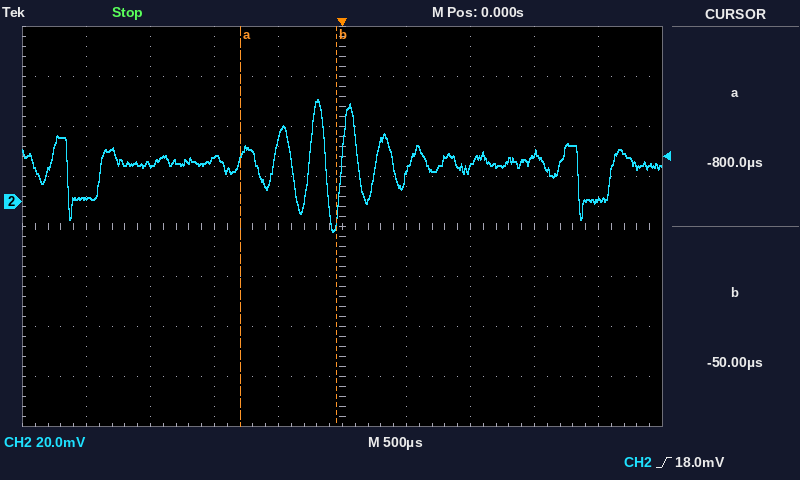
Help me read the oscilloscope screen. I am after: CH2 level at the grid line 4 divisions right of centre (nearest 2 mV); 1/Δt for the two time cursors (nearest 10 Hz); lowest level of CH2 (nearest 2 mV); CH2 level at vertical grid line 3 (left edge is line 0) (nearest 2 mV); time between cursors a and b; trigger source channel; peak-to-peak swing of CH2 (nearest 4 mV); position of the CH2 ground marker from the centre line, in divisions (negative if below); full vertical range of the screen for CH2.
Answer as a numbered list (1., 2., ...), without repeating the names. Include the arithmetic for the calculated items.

1. 0 mV
2. 1 / 750 µs ≈ 1.33 kHz
3. -12 mV
4. 18 mV
5. -50 µs − (-800 µs) = 750 µs
6. CH2
7. 52 mV
8. +0.5 div
9. 160 mV
